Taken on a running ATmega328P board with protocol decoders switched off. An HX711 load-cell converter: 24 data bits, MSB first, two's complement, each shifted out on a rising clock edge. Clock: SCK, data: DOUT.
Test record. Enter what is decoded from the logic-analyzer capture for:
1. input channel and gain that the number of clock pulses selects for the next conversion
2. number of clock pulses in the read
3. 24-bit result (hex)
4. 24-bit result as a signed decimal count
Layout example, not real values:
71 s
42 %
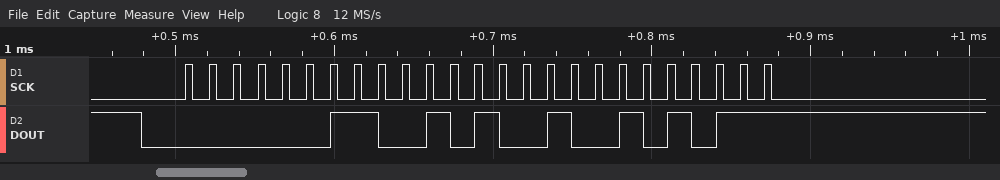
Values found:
channel A, gain 128
25
0x03292B
207147
